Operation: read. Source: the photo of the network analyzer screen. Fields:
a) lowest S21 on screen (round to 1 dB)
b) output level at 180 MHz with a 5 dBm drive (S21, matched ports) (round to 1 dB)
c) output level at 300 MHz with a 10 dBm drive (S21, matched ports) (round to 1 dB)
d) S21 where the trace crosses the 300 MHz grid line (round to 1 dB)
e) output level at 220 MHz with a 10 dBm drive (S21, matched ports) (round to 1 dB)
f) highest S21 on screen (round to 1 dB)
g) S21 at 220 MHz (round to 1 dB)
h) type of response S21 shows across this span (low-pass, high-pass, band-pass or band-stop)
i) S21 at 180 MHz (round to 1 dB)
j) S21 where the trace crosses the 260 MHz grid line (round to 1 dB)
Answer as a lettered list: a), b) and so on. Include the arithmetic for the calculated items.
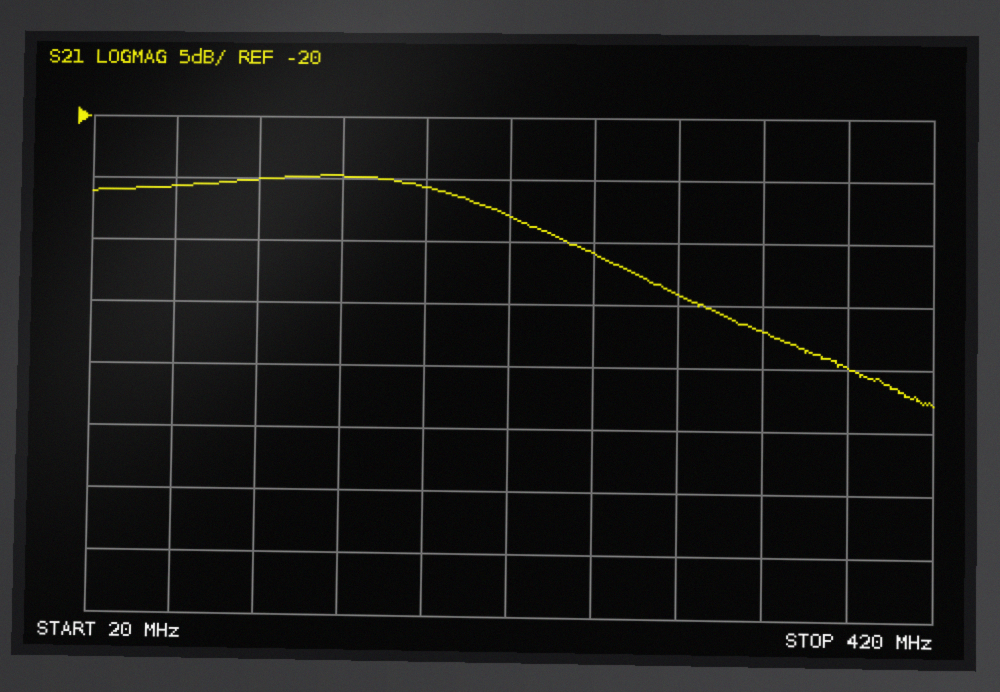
a) -43 dB
b) 5 dBm + (-26 dB) = -21 dBm
c) 10 dBm + (-34 dB) = -24 dBm
d) -34 dB
e) 10 dBm + (-28 dB) = -18 dBm
f) -25 dB
g) -28 dB
h) low-pass
i) -26 dB
j) -31 dB
